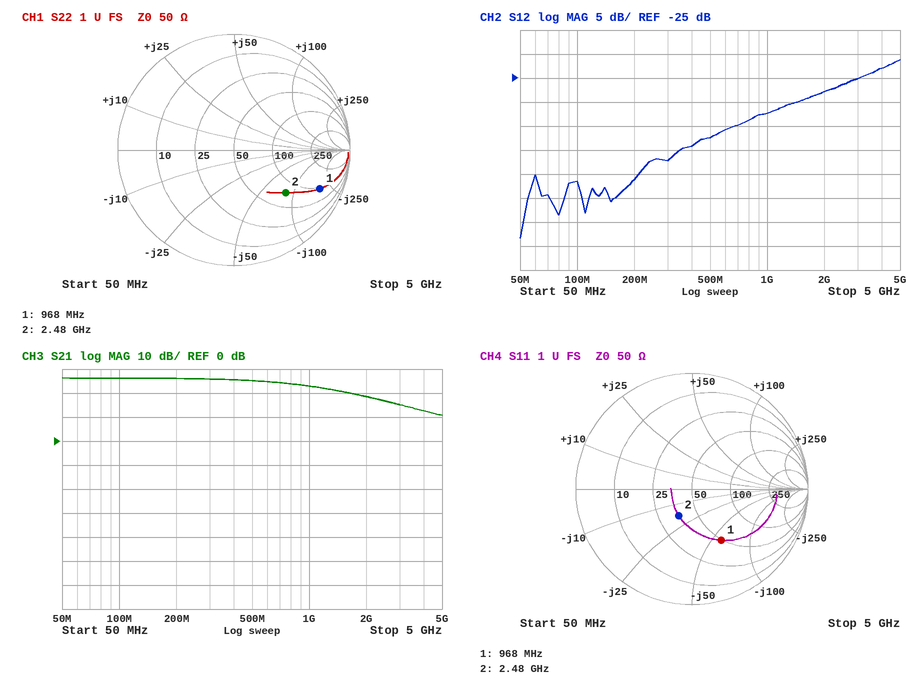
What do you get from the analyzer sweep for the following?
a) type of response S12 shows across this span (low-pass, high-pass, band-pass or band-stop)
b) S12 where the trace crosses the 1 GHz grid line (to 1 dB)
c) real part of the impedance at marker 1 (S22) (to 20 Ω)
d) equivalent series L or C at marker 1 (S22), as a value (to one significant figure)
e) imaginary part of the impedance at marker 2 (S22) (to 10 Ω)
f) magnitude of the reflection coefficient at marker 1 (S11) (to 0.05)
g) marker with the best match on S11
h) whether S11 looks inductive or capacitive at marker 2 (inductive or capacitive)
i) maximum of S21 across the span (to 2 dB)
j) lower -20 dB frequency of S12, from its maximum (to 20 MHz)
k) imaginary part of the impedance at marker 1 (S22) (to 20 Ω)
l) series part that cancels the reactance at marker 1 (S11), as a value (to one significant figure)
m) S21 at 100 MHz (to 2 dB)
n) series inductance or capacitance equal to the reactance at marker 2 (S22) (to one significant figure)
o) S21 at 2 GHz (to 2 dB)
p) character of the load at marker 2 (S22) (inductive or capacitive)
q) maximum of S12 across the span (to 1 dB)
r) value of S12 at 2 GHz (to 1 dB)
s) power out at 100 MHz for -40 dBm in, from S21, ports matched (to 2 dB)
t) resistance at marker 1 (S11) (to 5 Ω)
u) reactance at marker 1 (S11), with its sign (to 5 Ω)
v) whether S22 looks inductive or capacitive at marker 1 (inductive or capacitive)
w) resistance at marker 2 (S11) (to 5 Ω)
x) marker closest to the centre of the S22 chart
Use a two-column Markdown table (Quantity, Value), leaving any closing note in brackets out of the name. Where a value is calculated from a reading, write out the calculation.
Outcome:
| Quantity | Value |
|---|---|
| type of response S12 shows across this span | high-pass |
| S12 where the trace crosses the 1 GHz grid line | -32 dB |
| real part of the impedance at marker 1 (S22) | 100 Ω |
| equivalent series L or C at marker 1 (S22), as a value | C = 1/(2π × 968 MHz × 180 Ω) ≈ 913 fF, so 900 fF to one significant figure |
| imaginary part of the impedance at marker 2 (S22) | -80 Ω |
| magnitude of the reflection coefficient at marker 1 (S11) | 0.50 |
| marker with the best match on S11 | marker 2 |
| whether S11 looks inductive or capacitive at marker 2 | capacitive |
| maximum of S21 across the span | 26 dB |
| lower -20 dB frequency of S12, from its maximum | 320 MHz |
| imaginary part of the impedance at marker 1 (S22) | -180 Ω |
| series part that cancels the reactance at marker 1 (S11), as a value | L = 60 Ω/(2π × 968 MHz) ≈ 10 nH |
| S21 at 100 MHz | 26 dB |
| series inductance or capacitance equal to the reactance at marker 2 (S22) | C = 1/(2π × 2.48 GHz × 80 Ω) ≈ 802 fF, so 800 fF to one significant figure |
| S21 at 2 GHz | 18 dB |
| character of the load at marker 2 (S22) | capacitive |
| maximum of S12 across the span | -21 dB |
| value of S12 at 2 GHz | -28 dB |
| power out at 100 MHz for -40 dBm in, from S21, ports matched | -40 dBm + (26 dB) = -14 dBm |
| resistance at marker 1 (S11) | 50 Ω |
| reactance at marker 1 (S11), with its sign | -60 Ω |
| whether S22 looks inductive or capacitive at marker 1 | capacitive |
| resistance at marker 2 (S11) | 35 Ω |
| marker closest to the centre of the S22 chart | marker 2 |
